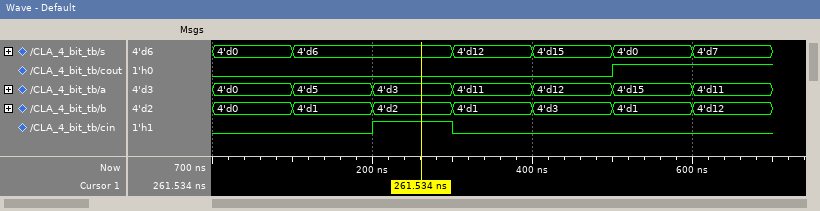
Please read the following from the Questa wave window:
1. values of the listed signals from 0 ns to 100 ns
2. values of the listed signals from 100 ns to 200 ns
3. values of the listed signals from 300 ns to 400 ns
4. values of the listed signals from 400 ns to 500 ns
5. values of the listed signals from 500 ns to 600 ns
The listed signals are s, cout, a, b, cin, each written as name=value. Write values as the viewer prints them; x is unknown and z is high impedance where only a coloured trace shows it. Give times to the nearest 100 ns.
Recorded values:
s=4'd0, cout=0, a=4'd0, b=4'd0, cin=0
s=4'd6, cout=0, a=4'd5, b=4'd1, cin=0
s=4'd12, cout=0, a=4'd11, b=4'd1, cin=0
s=4'd15, cout=0, a=4'd12, b=4'd3, cin=0
s=4'd0, cout=1, a=4'd15, b=4'd1, cin=0
